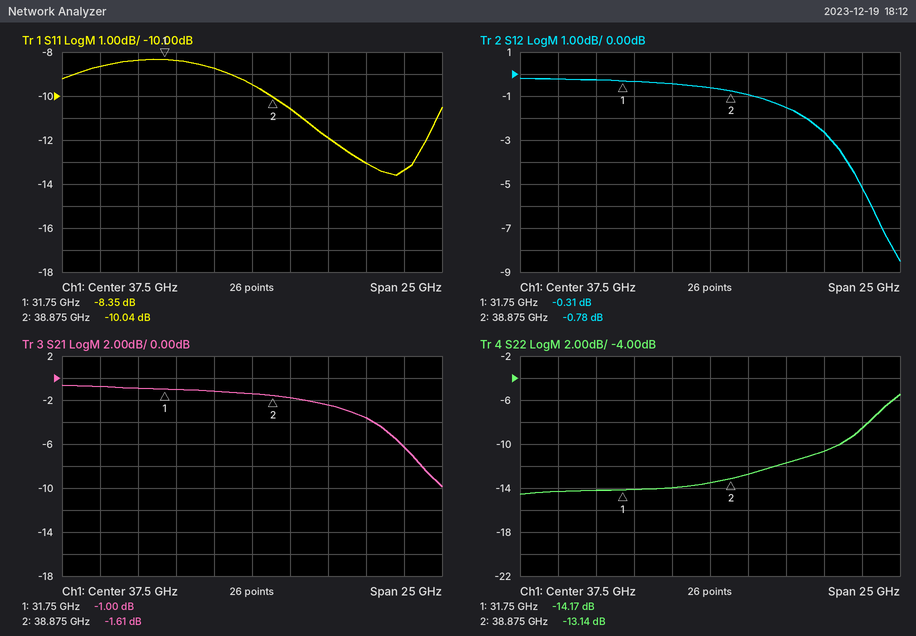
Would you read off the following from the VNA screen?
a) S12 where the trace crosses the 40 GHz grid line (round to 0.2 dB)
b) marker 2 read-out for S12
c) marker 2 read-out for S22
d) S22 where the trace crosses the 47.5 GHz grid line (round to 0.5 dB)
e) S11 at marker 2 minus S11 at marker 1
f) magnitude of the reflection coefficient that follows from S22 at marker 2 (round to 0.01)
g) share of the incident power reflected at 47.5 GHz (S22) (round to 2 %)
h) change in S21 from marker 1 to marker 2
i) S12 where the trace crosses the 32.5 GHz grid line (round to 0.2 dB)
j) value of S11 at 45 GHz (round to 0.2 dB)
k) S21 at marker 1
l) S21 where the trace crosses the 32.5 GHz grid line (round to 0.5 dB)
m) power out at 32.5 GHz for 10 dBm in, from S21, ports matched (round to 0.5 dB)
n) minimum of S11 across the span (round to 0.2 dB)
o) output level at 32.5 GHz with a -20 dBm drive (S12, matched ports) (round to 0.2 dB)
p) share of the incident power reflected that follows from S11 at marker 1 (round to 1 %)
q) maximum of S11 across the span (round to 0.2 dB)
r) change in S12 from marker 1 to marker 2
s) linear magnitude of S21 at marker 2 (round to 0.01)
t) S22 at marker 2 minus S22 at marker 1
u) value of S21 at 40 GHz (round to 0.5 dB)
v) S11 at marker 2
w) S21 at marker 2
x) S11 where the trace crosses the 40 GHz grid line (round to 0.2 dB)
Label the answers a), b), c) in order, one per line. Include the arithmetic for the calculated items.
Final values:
a) -1.0 dB
b) -0.78 dB
c) -13.14 dB
d) -8.5 dB
e) -10.04 − (-8.35) = -1.69 dB
f) 10^(-13.14/20) ≈ 0.22
g) 10^(-8.5/10) ≈ 14 %
h) -1.61 − (-1) = -0.61 dB
i) -0.4 dB
j) -13.0 dB
k) -1.00 dB
l) -1.0 dB
m) 10 dBm + (-1.0 dB) = 9.0 dBm
n) -13.6 dB
o) -20 dBm + (-0.4 dB) = -20.4 dBm
p) 10^(-8.35/10) ≈ 15 %
q) -8.4 dB
r) -0.78 − (-0.31) = -0.47 dB
s) 10^(-1.61/20) ≈ 0.83
t) -13.14 − (-14.17) = 1.03 dB
u) -2.0 dB
v) -10.04 dB
w) -1.61 dB
x) -10.6 dB
